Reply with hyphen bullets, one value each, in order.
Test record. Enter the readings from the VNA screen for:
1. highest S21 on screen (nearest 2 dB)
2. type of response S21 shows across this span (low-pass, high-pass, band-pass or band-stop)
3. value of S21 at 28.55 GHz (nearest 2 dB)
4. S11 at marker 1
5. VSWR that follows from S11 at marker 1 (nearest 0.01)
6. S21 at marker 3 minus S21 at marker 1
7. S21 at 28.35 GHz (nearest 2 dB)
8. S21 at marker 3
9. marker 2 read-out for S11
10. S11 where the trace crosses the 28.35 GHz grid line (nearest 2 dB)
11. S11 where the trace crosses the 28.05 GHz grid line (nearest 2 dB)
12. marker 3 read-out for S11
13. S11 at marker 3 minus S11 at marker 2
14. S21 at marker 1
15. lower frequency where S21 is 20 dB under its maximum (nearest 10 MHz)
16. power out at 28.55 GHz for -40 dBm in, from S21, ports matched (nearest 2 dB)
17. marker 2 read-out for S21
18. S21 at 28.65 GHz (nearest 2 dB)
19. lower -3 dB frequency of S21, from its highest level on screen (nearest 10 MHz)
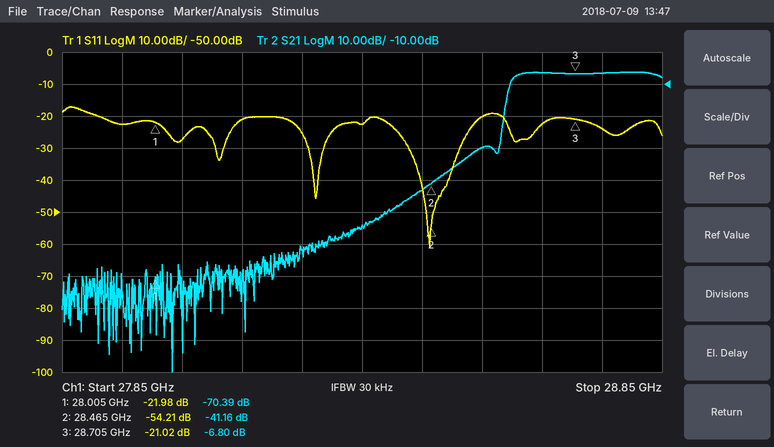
- -6 dB
- high-pass
- -30 dB
- -21.98 dB
- 1.17
- 63.59 dB
- -54 dB
- -6.80 dB
- -54.21 dB
- -22 dB
- -28 dB
- -21.02 dB
- 33.19 dB
- -70.39 dB
- 28.58 GHz
- -70 dBm
- -41.16 dB
- -6 dB
- 28.60 GHz
